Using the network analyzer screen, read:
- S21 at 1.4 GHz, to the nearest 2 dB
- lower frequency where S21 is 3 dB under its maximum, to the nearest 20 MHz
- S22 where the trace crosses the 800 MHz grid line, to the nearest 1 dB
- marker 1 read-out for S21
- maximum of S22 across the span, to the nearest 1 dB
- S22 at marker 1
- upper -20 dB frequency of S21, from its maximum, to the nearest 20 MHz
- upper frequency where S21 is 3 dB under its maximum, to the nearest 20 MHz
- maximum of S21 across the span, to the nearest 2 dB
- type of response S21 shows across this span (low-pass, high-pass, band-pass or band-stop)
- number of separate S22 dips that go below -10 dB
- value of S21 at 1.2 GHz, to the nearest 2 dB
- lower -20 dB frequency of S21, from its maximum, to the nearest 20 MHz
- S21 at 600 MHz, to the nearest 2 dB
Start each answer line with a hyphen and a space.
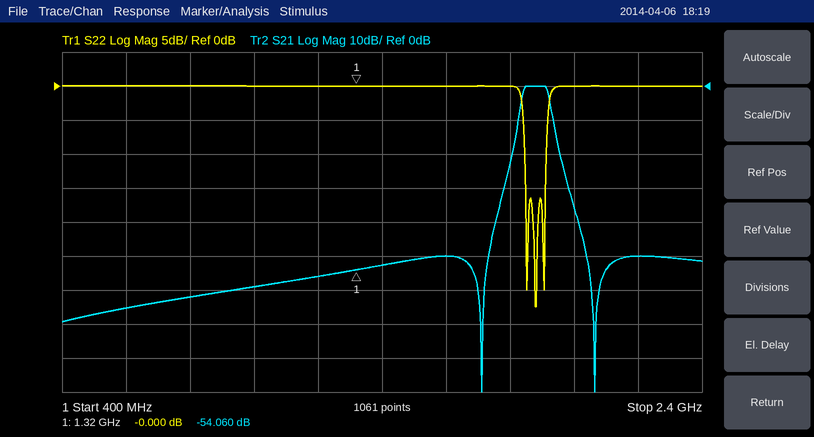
- -52 dB
- 1.84 GHz
- 0 dB
- -54.060 dB
- 0 dB
- -0.000 dB
- 1.96 GHz
- 1.92 GHz
- 0 dB
- band-pass
- 3
- -56 dB
- 1.80 GHz
- -66 dB
